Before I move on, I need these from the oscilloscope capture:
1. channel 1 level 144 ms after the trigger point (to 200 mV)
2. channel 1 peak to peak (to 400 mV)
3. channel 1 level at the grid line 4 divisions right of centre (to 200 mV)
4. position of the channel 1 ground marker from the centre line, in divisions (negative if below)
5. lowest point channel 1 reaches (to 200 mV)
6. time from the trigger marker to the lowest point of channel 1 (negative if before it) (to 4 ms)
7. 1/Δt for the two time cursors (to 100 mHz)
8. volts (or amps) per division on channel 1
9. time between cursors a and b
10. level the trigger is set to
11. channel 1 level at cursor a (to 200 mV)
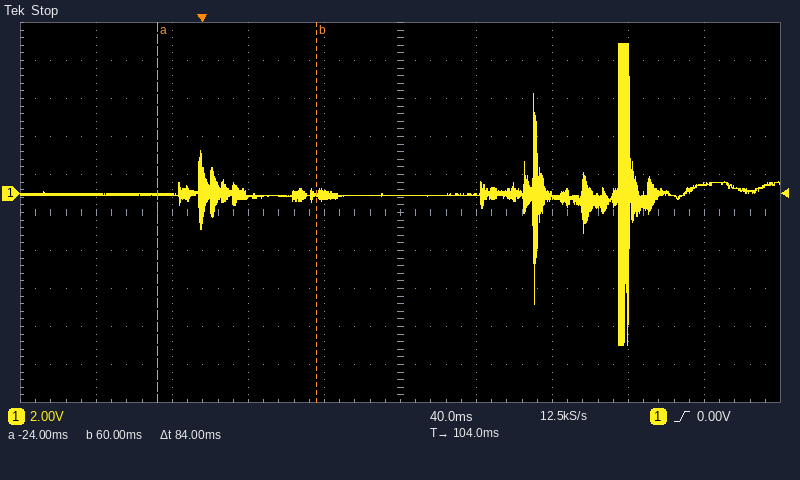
0.0 V
16.0 V
400 mV
+0.5 div
-8.0 V
+220 ms
11.9 Hz
2 V
84 ms
0.00 V
0.0 V
